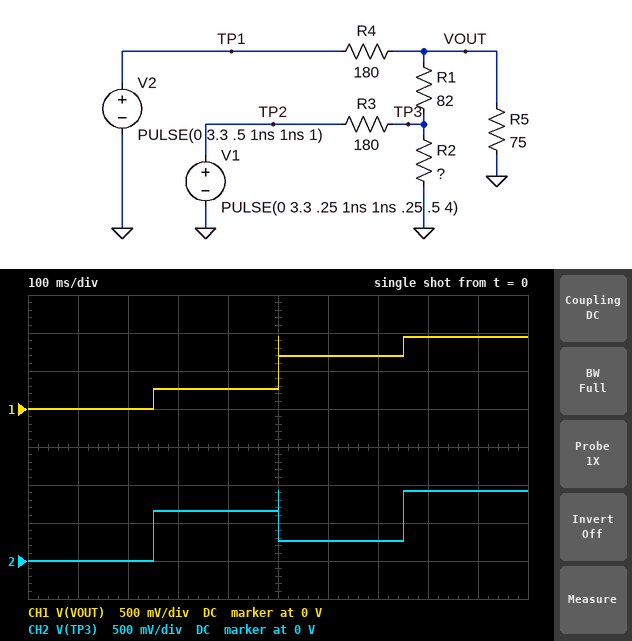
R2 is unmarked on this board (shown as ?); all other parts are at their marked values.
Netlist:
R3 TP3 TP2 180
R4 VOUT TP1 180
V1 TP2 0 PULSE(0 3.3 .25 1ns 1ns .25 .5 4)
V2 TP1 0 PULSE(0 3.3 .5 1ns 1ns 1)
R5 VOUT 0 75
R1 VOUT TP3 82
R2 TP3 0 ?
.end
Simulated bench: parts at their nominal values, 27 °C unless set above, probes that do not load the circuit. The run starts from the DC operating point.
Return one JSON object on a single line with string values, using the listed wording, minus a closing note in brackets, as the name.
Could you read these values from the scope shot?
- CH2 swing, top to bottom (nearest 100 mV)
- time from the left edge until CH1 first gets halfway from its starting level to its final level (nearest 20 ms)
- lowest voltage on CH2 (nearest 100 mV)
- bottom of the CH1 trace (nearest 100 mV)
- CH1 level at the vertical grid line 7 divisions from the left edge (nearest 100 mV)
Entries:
{"CH2 swing, top to bottom": "900 mV", "time from the left edge until CH1 first gets halfway from its starting level to its final level": "500 ms", "lowest voltage on CH2": "0 V", "bottom of the CH1 trace": "0 V", "CH1 level at the vertical grid line 7 divisions from the left edge": "700 mV"}
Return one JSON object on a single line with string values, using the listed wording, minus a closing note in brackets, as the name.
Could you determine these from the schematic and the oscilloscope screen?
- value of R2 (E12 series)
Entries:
{"value of R2": "68 Ω"}
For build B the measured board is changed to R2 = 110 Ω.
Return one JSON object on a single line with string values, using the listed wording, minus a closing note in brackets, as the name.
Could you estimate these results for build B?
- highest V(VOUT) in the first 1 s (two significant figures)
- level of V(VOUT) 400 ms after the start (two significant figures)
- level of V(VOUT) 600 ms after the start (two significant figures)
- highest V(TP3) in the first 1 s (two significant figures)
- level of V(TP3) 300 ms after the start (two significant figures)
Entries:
{"highest V(VOUT) in the first 1 s": "1.0 V", "level of V(VOUT) 400 ms after the start": "330 mV", "level of V(VOUT) 600 ms after the start": "720 mV", "highest V(TP3) in the first 1 s": "1.2 V", "level of V(TP3) 300 ms after the start": "830 mV"}
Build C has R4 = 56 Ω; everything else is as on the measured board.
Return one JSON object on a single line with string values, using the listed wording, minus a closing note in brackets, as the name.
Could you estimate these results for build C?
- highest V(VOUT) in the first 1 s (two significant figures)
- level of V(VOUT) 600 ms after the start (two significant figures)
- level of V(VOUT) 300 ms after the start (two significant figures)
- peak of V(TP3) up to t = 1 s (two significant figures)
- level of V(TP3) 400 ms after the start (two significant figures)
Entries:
{"highest V(VOUT) in the first 1 s": "1.7 V", "level of V(VOUT) 600 ms after the start": "1.5 V", "level of V(VOUT) 300 ms after the start": "180 mV", "peak of V(TP3) up to t = 1 s": "1.2 V", "level of V(TP3) 400 ms after the start": "630 mV"}
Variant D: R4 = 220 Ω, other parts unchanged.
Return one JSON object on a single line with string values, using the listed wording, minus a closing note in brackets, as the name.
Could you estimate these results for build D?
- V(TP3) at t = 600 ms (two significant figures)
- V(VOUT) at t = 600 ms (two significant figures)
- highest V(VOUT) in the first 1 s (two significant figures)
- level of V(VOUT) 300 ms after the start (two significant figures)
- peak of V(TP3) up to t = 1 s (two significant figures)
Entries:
{"V(TP3) at t = 600 ms": "220 mV", "V(VOUT) at t = 600 ms": "590 mV", "highest V(VOUT) in the first 1 s": "860 mV", "level of V(VOUT) 300 ms after the start": "270 mV", "peak of V(TP3) up to t = 1 s": "890 mV"}
